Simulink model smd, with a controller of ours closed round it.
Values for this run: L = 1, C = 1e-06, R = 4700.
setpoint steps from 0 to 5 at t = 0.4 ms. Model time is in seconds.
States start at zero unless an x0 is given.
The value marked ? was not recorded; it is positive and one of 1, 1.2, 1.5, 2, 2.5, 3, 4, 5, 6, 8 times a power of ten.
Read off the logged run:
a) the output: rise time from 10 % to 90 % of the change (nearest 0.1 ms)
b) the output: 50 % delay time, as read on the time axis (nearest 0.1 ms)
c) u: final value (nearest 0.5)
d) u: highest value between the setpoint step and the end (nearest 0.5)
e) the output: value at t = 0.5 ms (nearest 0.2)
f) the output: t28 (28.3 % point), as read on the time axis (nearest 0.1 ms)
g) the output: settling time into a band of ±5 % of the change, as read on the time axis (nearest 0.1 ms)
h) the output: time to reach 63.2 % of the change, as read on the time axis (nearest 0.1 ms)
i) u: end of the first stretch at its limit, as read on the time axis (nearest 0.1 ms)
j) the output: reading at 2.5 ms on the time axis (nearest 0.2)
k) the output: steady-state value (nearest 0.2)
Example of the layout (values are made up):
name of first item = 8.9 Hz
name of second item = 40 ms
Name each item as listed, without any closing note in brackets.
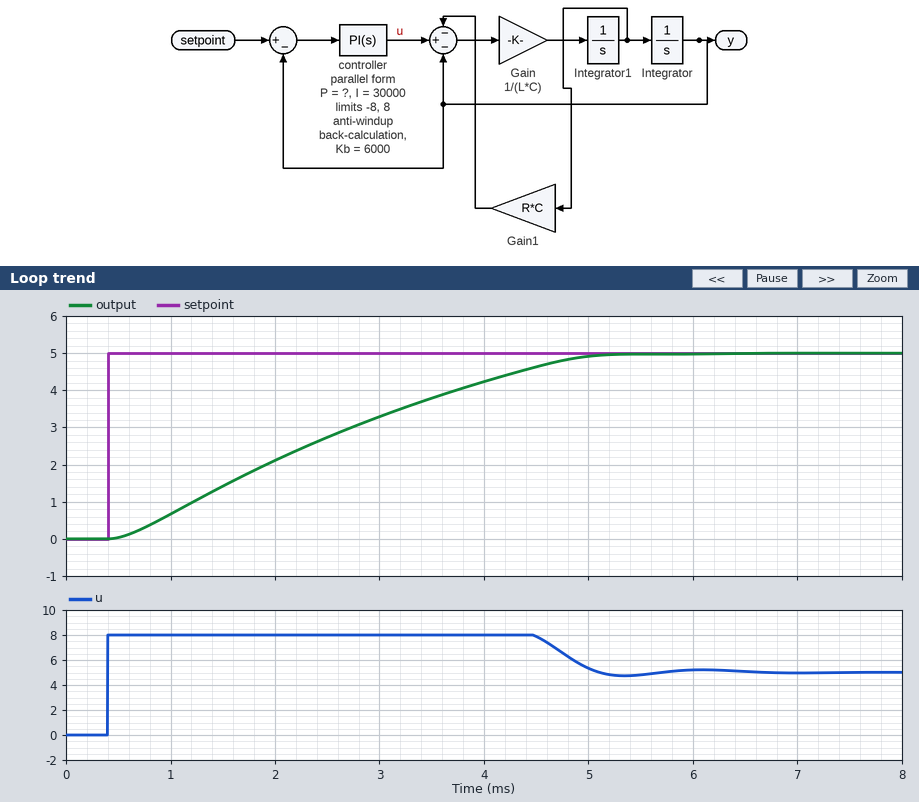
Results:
the output: rise time from 10 % to 90 % of the change = 3.4 ms
the output: 50 % delay time, as read on the time axis = 2.3 ms
u: final value = 5.0
u: highest value between the setpoint step and the end = 8.0
the output: value at t = 0.5 ms = 0.0
the output: t28 (28.3 % point), as read on the time axis = 1.5 ms
the output: settling time into a band of ±5 % of the change, as read on the time axis = 4.7 ms
the output: time to reach 63.2 % of the change, as read on the time axis = 2.9 ms
u: end of the first stretch at its limit, as read on the time axis = 4.5 ms
the output: reading at 2.5 ms on the time axis = 2.8
the output: steady-state value = 5.0
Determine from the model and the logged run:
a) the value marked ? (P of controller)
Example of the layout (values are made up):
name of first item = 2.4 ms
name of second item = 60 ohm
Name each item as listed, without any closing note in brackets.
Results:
the value marked ? = 20
